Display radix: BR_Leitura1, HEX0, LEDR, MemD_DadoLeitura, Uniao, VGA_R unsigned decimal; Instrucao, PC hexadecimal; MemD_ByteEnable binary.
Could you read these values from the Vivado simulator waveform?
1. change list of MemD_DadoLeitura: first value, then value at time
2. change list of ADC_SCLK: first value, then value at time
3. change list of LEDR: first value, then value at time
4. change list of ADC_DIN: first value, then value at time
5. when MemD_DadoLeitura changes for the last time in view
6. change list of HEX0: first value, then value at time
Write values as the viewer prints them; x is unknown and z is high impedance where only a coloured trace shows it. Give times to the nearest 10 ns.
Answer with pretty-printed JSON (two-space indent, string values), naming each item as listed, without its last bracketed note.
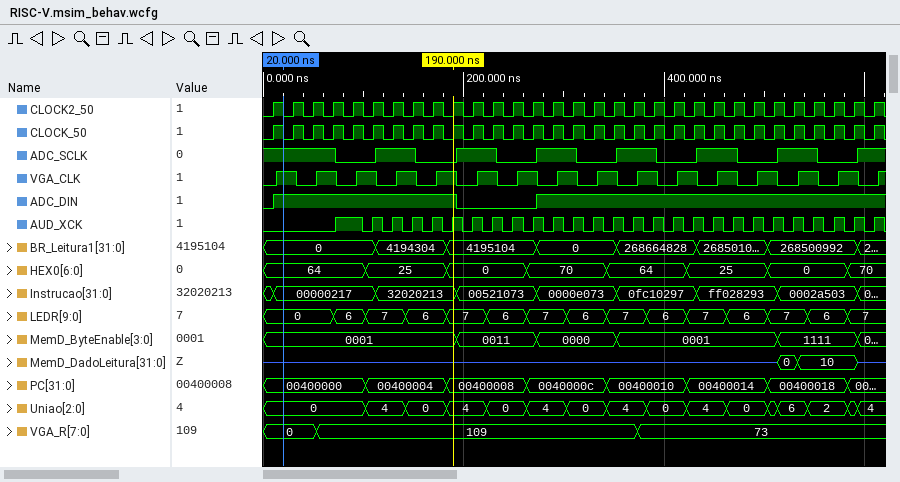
{
  "change list of MemD_DadoLeitura: first value, then value at time": "z, 0 at 510 ns, 10 at 530 ns, z at 590 ns",
  "change list of ADC_SCLK: first value, then value at time": "1, 0 at 70 ns, 1 at 110 ns, 0 at 150 ns, 1 at 190 ns, 0 at 230 ns, 1 at 270 ns, 0 at 310 ns, 1 at 350 ns, 0 at 390 ns, 1 at 430 ns, 0 at 470 ns, 1 at 510 ns, 0 at 550 ns, 1 at 590 ns",
  "change list of LEDR: first value, then value at time": "0, 6 at 70 ns, 7 at 100 ns, 6 at 140 ns, 7 at 180 ns, 6 at 220 ns, 7 at 260 ns, 6 at 300 ns, 7 at 340 ns, 6 at 380 ns, 7 at 420 ns, 6 at 460 ns, 7 at 500 ns, 6 at 540 ns, 7 at 580 ns",
  "change list of ADC_DIN: first value, then value at time": "0, 1 at 10 ns, 0 at 190 ns, 1 at 270 ns",
  "when MemD_DadoLeitura changes for the last time in view": "590 ns",
  "change list of HEX0: first value, then value at time": "64, 25 at 100 ns, 0 at 180 ns, 70 at 260 ns, 64 at 340 ns, 25 at 420 ns, 0 at 500 ns, 70 at 580 ns"
}
